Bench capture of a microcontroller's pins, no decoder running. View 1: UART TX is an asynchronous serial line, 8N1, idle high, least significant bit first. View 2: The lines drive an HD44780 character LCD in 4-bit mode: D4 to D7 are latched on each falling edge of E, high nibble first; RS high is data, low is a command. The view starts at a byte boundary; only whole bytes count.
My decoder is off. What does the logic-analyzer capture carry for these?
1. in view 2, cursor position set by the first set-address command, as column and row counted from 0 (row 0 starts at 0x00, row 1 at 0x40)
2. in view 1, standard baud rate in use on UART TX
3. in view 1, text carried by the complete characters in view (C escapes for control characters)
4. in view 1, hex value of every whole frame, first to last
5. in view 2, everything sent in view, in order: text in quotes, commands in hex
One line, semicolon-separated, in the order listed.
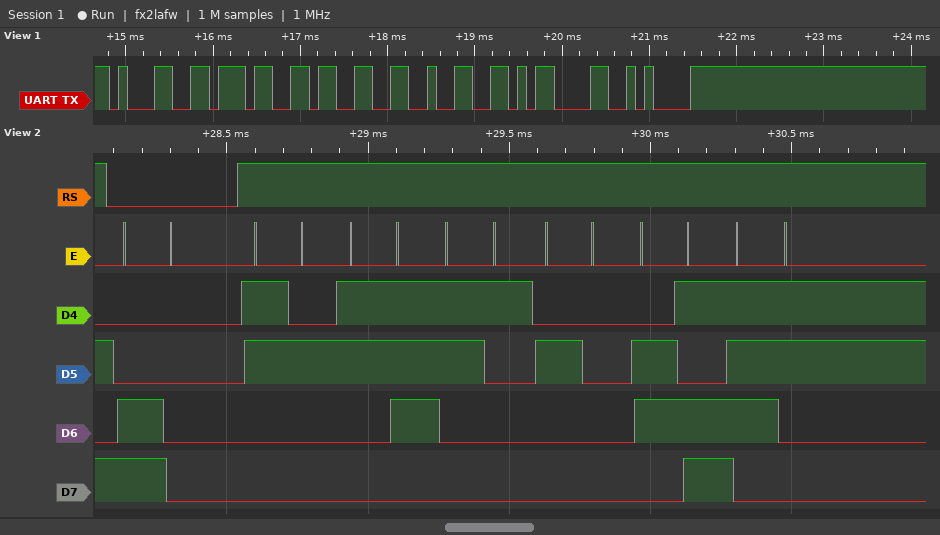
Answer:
column 0, row 1; 9600 baud; "1732\r\n"; 31 37 33 32 0D 0A; 0xC0 "271 ms"
